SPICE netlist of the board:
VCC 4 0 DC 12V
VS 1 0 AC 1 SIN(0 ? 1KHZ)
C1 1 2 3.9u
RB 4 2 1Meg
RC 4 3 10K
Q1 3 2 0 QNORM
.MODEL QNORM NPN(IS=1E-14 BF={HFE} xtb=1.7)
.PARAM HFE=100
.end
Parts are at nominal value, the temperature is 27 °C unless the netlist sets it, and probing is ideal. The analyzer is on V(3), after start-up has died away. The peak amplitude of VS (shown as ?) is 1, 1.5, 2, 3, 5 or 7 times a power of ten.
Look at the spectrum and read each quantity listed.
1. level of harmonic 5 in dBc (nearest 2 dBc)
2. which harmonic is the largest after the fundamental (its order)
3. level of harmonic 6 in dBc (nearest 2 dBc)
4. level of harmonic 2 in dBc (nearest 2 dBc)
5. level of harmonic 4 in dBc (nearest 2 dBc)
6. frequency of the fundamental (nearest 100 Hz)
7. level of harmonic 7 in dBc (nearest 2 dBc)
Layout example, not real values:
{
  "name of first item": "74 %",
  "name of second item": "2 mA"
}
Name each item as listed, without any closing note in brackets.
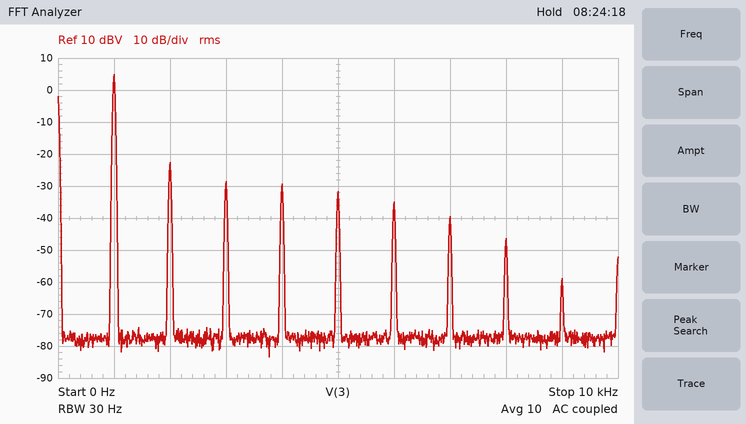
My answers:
{
  "level of harmonic 5 in dBc": "-36 dBc",
  "which harmonic is the largest after the fundamental": "2",
  "level of harmonic 6 in dBc": "-40 dBc",
  "level of harmonic 2 in dBc": "-28 dBc",
  "level of harmonic 4 in dBc": "-34 dBc",
  "frequency of the fundamental": "1.0 kHz",
  "level of harmonic 7 in dBc": "-44 dBc"
}
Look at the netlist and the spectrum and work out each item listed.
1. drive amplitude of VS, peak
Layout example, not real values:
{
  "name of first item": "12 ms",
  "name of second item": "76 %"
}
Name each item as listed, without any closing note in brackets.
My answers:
{
  "drive amplitude of VS, peak": "7 mV"
}
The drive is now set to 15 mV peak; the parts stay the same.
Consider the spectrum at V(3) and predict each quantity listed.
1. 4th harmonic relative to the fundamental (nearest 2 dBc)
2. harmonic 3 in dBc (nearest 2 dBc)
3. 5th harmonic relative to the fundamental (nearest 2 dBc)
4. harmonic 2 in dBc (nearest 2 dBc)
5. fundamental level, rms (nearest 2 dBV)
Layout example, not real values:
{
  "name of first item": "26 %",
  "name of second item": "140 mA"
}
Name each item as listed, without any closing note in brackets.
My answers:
{
  "4th harmonic relative to the fundamental": "-32 dBc",
  "harmonic 3 in dBc": "-36 dBc",
  "5th harmonic relative to the fundamental": "-34 dBc",
  "harmonic 2 in dBc": "-18 dBc",
  "fundamental level, rms": "10 dBV"
}
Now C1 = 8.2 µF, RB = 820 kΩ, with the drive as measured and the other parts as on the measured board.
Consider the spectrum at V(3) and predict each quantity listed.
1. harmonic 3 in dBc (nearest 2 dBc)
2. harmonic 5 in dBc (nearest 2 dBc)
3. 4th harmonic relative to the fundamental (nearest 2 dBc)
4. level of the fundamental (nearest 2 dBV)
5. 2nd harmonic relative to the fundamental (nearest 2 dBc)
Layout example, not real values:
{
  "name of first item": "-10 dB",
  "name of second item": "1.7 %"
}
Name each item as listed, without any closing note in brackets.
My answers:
{
  "harmonic 3 in dBc": "-28 dBc",
  "harmonic 5 in dBc": "-34 dBc",
  "4th harmonic relative to the fundamental": "-30 dBc",
  "level of the fundamental": "4 dBV",
  "2nd harmonic relative to the fundamental": "-36 dBc"
}
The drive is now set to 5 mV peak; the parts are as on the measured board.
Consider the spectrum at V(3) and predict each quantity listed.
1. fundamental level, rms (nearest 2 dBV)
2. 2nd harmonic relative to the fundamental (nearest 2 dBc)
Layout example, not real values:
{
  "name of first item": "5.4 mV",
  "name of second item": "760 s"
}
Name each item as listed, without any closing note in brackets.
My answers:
{
  "fundamental level, rms": "2 dBV",
  "2nd harmonic relative to the fundamental": "-32 dBc"
}
